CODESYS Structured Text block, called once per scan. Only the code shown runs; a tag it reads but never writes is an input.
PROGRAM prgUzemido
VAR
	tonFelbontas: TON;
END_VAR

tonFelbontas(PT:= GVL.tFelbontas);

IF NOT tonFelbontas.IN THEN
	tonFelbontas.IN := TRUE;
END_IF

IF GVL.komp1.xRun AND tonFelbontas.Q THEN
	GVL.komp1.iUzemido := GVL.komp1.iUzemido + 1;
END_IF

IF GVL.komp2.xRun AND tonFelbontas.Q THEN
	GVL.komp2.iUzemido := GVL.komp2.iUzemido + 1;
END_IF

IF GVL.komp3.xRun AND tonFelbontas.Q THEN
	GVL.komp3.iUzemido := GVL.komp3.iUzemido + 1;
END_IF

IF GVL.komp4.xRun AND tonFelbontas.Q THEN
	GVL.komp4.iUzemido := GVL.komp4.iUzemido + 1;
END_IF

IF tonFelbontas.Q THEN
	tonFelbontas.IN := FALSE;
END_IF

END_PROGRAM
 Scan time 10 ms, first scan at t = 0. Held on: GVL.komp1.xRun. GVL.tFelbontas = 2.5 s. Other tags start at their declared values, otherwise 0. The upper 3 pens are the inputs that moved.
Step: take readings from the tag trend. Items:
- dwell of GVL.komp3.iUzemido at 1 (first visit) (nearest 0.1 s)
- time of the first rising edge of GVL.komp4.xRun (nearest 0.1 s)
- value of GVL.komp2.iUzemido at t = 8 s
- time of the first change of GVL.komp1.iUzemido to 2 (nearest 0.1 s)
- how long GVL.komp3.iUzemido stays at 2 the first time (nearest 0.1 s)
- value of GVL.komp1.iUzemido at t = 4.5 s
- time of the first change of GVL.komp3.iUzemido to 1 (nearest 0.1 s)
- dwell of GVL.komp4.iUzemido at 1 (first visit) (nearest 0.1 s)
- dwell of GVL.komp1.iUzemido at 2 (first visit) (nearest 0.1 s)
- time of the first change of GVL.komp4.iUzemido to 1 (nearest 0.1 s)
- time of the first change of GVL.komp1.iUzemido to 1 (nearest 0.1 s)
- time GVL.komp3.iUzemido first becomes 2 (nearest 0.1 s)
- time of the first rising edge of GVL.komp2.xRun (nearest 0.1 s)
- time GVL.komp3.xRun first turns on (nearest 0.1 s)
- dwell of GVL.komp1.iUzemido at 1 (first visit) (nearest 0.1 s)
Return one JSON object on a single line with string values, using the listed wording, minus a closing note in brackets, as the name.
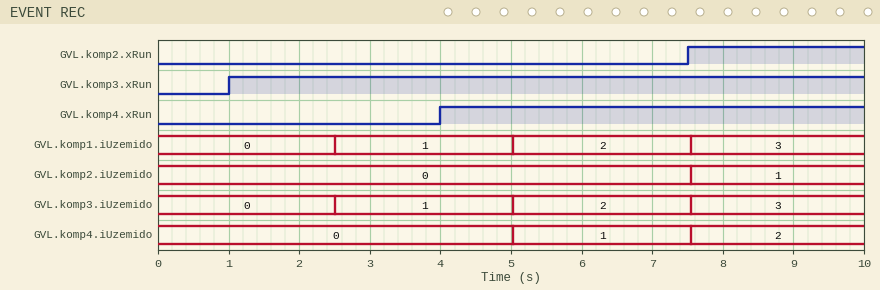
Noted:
{"dwell of GVL.komp3.iUzemido at 1 (first visit)": "2.5 s", "time of the first rising edge of GVL.komp4.xRun": "4.0 s", "value of GVL.komp2.iUzemido at t = 8 s": "1", "time of the first change of GVL.komp1.iUzemido to 2": "5.0 s", "how long GVL.komp3.iUzemido stays at 2 the first time": "2.5 s", "value of GVL.komp1.iUzemido at t = 4.5 s": "1", "time of the first change of GVL.komp3.iUzemido to 1": "2.5 s", "dwell of GVL.komp4.iUzemido at 1 (first visit)": "2.5 s", "dwell of GVL.komp1.iUzemido at 2 (first visit)": "2.5 s", "time of the first change of GVL.komp4.iUzemido to 1": "5.0 s", "time of the first change of GVL.komp1.iUzemido to 1": "2.5 s", "time GVL.komp3.iUzemido first becomes 2": "5.0 s", "time of the first rising edge of GVL.komp2.xRun": "7.5 s", "time GVL.komp3.xRun first turns on": "1.0 s", "dwell of GVL.komp1.iUzemido at 1 (first visit)": "2.5 s"}
